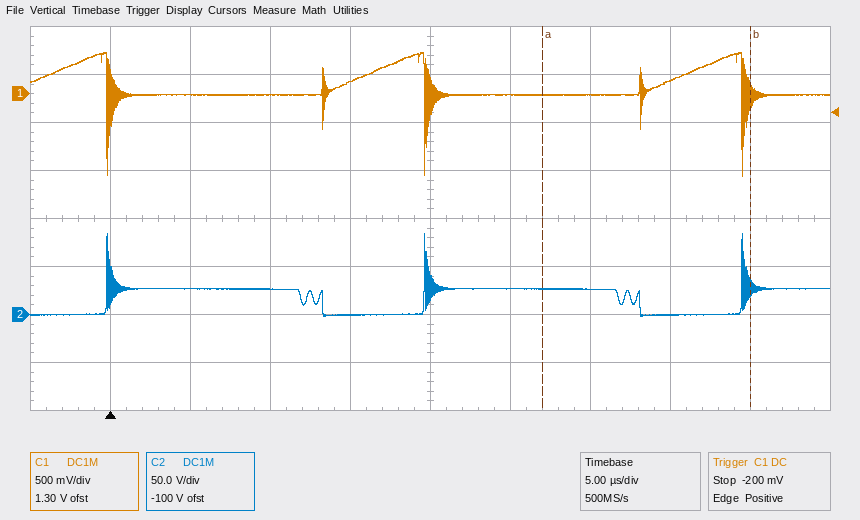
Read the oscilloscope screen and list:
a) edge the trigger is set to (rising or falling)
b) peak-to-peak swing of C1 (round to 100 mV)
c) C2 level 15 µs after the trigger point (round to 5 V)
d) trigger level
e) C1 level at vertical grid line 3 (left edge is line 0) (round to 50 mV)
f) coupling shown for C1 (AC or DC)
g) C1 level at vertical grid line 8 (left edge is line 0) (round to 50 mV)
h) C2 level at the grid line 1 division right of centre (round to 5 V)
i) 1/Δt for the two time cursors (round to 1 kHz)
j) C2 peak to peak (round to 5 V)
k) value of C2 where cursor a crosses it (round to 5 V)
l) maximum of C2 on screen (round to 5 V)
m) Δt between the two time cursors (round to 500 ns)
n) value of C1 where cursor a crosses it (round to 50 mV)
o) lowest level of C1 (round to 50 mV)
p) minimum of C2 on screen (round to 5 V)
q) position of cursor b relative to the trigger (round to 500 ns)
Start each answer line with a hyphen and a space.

- rising
- 1.30 V
- 0 V
- -200 mV
- 0 mV
- DC
- 150 mV
- 25 V
- 77 kHz
- 85 V
- 25 V
- 85 V
- 13.0 µs
- 0 mV
- -850 mV
- 0 V
- +40.0 µs
